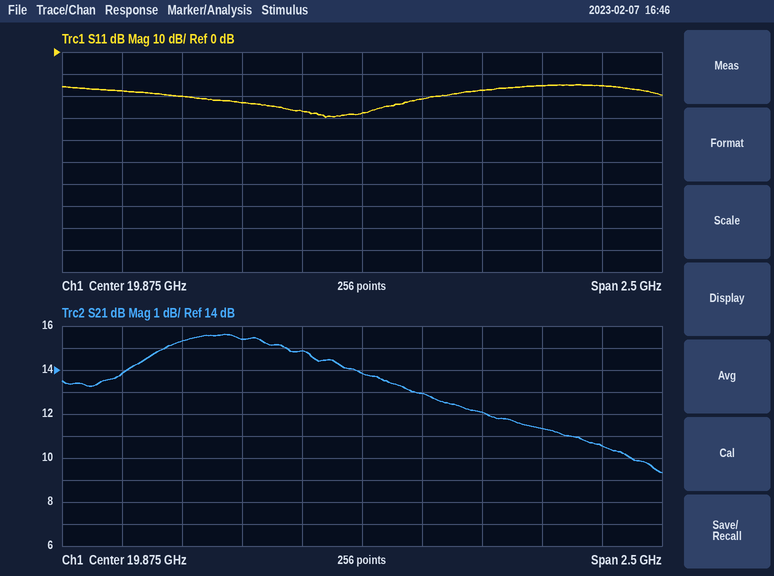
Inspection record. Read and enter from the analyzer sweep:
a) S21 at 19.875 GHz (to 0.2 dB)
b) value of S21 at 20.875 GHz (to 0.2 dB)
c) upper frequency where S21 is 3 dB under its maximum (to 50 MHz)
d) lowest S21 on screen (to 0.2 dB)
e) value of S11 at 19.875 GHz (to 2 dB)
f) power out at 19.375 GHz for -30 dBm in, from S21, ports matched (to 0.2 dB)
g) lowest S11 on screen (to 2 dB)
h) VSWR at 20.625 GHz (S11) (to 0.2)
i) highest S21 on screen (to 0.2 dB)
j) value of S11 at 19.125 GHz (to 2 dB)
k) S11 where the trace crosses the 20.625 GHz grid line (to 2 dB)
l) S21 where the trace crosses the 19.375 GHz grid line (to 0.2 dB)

13.8 dB
10.6 dB
20.20 GHz
9.4 dB
-28 dB
-14.6 dBm
-30 dB
1.4
15.6 dB
-20 dB
-16 dB
15.4 dB
